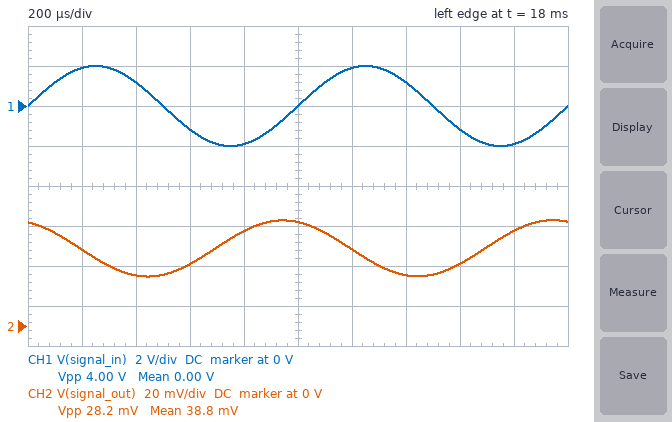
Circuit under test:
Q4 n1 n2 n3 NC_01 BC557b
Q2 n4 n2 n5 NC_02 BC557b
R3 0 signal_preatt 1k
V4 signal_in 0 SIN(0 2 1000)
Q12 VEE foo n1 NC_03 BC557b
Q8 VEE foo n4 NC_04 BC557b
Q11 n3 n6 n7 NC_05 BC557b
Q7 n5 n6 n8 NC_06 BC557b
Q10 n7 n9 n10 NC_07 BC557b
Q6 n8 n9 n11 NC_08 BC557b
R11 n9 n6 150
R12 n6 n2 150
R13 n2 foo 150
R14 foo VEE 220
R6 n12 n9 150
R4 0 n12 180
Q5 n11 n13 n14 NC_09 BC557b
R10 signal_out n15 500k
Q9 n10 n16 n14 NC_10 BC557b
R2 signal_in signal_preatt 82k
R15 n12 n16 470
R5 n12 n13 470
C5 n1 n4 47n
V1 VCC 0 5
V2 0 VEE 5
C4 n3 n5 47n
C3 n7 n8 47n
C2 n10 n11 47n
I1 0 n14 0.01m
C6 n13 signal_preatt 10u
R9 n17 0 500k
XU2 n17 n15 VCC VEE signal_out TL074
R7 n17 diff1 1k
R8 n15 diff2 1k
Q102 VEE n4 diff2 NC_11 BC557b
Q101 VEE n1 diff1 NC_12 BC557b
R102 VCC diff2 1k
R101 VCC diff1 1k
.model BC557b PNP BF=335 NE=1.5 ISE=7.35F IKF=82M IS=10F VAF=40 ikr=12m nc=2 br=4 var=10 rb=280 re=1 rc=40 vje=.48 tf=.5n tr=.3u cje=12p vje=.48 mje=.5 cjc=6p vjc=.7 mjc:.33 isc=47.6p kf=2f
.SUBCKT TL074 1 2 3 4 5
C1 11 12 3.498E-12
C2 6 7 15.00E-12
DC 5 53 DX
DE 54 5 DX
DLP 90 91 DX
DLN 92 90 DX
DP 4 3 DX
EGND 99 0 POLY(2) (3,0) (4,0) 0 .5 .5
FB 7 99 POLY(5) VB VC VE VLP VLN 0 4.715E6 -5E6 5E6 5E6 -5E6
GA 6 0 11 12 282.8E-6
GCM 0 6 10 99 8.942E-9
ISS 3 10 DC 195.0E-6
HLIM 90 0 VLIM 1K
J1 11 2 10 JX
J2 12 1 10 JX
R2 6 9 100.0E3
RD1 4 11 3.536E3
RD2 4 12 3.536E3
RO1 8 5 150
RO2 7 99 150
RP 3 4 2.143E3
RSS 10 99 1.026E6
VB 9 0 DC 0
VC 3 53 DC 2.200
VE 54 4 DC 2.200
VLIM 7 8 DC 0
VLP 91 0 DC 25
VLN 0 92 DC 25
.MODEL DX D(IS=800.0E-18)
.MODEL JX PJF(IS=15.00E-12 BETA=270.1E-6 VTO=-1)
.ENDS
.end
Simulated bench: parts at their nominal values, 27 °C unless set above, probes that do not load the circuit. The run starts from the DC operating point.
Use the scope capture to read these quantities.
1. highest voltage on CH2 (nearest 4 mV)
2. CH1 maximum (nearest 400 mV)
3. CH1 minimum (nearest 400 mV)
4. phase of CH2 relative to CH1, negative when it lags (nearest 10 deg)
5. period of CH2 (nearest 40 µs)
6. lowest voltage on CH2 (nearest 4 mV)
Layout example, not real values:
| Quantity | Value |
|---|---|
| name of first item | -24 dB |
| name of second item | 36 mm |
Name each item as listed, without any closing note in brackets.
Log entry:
| Quantity | Value |
|---|---|
| highest voltage on CH2 | 52 mV |
| CH1 maximum | 2.0 V |
| CH1 minimum | -2.0 V |
| phase of CH2 relative to CH1, negative when it lags | 110 deg |
| period of CH2 | 1.00 ms |
| lowest voltage on CH2 | 24 mV |
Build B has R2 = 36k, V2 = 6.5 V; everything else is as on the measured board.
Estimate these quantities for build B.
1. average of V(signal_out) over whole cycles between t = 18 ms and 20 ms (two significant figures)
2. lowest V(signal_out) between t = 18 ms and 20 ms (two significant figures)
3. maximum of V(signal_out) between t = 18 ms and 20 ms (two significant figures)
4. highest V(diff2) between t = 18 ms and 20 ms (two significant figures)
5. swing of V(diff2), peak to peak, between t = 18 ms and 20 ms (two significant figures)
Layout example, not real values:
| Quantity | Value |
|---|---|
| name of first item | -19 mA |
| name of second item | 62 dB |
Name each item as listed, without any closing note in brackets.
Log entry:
| Quantity | Value |
|---|---|
| average of V(signal_out) over whole cycles between t = 18 ms and 20 ms | 41 mV |
| lowest V(signal_out) between t = 18 ms and 20 ms | 13 mV |
| maximum of V(signal_out) between t = 18 ms and 20 ms | 69 mV |
| highest V(diff2) between t = 18 ms and 20 ms | -3.8 V |
| swing of V(diff2), peak to peak, between t = 18 ms and 20 ms | 2.7 mV |
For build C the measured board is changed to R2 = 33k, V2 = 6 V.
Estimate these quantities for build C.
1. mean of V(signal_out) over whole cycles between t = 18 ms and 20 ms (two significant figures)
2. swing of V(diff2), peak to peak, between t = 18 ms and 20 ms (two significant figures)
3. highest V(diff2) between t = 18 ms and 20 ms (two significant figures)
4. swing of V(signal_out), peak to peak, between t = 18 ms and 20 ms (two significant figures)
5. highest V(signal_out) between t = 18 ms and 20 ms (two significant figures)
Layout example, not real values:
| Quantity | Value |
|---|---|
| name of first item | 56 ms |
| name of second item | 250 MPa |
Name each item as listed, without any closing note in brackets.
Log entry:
| Quantity | Value |
|---|---|
| mean of V(signal_out) over whole cycles between t = 18 ms and 20 ms | 39 mV |
| swing of V(diff2), peak to peak, between t = 18 ms and 20 ms | 2.9 mV |
| highest V(diff2) between t = 18 ms and 20 ms | -3.4 V |
| swing of V(signal_out), peak to peak, between t = 18 ms and 20 ms | 63 mV |
| highest V(signal_out) between t = 18 ms and 20 ms | 71 mV |
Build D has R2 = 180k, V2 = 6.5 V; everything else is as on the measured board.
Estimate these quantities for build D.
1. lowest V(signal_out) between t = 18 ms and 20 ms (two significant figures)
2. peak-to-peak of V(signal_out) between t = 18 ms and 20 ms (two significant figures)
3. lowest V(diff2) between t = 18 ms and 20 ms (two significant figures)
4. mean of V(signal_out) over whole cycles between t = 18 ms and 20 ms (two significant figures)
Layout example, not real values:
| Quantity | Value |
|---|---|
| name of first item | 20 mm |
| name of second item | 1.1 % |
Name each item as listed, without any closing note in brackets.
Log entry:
| Quantity | Value |
|---|---|
| lowest V(signal_out) between t = 18 ms and 20 ms | 38 mV |
| peak-to-peak of V(signal_out) between t = 18 ms and 20 ms | 12 mV |
| lowest V(diff2) between t = 18 ms and 20 ms | -3.8 V |
| mean of V(signal_out) over whole cycles between t = 18 ms and 20 ms | 44 mV |
